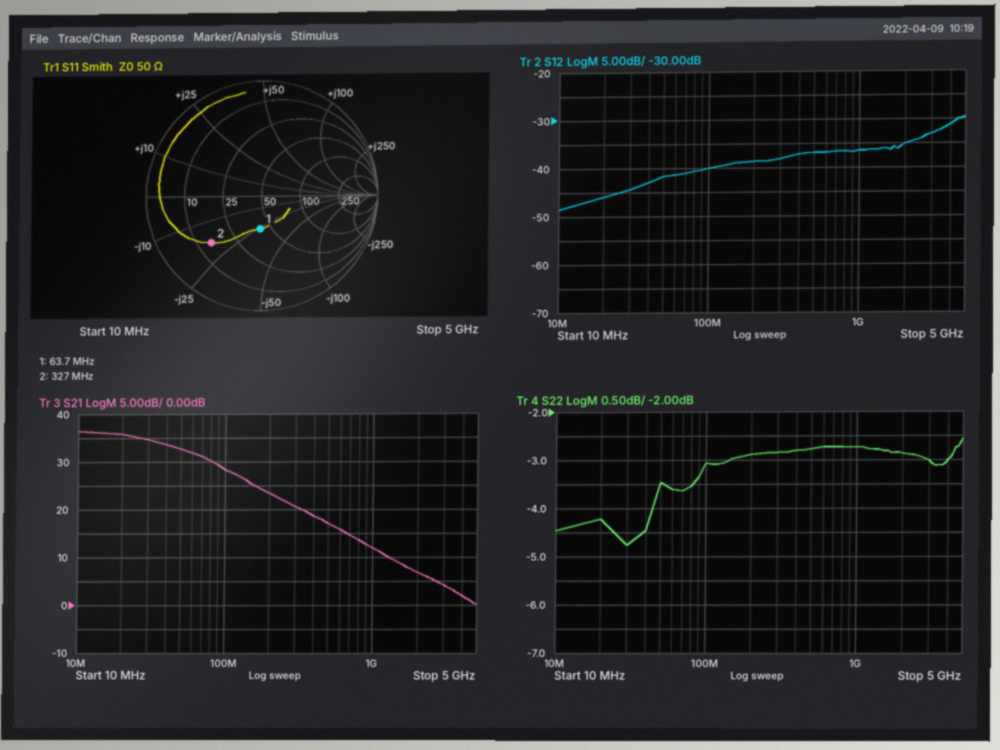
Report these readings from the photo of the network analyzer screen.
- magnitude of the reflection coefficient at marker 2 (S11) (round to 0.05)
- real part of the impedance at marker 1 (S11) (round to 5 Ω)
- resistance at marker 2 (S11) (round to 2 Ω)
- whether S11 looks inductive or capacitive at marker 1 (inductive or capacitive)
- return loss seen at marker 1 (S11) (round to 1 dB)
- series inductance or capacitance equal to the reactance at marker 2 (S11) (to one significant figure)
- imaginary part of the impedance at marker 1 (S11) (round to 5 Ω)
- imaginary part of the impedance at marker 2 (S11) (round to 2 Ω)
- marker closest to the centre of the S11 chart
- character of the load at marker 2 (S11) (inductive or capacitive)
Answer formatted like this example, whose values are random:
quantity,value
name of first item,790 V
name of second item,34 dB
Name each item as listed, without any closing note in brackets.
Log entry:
quantity,value
magnitude of the reflection coefficient at marker 2 (S11),0.60
real part of the impedance at marker 1 (S11),40 Ω
resistance at marker 2 (S11),14 Ω
whether S11 looks inductive or capacitive at marker 1,capacitive
return loss seen at marker 1 (S11),11 dB
series inductance or capacitance equal to the reactance at marker 2 (S11),30 pF
imaginary part of the impedance at marker 1 (S11),-25 Ω
imaginary part of the impedance at marker 2 (S11),-18 Ω
marker closest to the centre of the S11 chart,marker 1
character of the load at marker 2 (S11),capacitive
